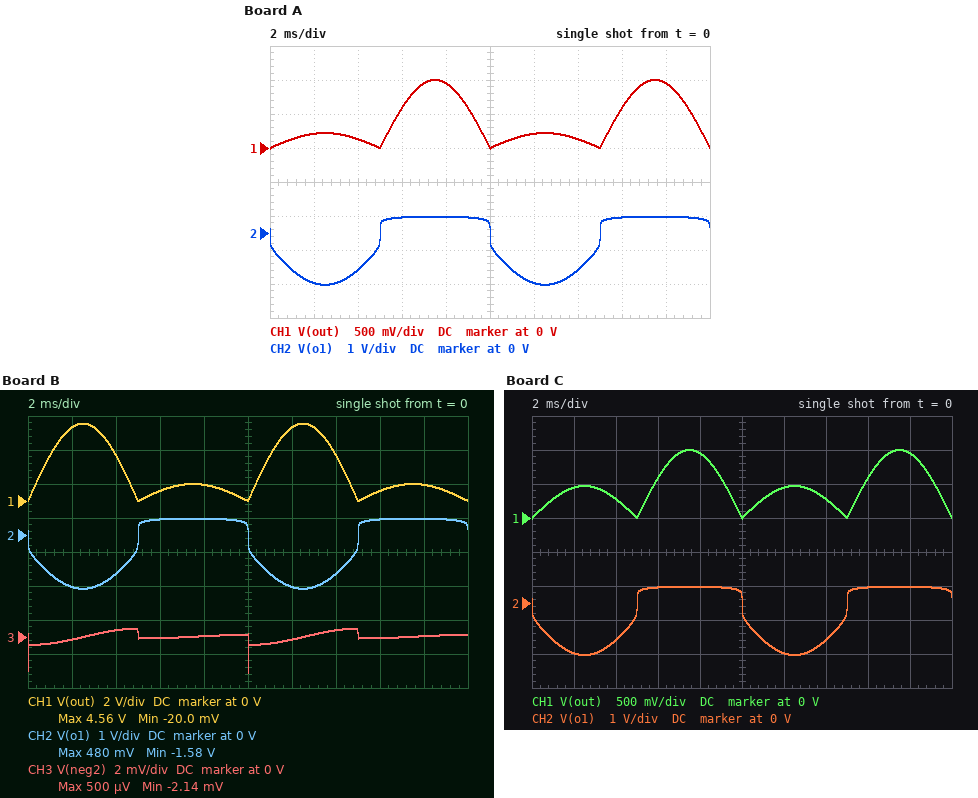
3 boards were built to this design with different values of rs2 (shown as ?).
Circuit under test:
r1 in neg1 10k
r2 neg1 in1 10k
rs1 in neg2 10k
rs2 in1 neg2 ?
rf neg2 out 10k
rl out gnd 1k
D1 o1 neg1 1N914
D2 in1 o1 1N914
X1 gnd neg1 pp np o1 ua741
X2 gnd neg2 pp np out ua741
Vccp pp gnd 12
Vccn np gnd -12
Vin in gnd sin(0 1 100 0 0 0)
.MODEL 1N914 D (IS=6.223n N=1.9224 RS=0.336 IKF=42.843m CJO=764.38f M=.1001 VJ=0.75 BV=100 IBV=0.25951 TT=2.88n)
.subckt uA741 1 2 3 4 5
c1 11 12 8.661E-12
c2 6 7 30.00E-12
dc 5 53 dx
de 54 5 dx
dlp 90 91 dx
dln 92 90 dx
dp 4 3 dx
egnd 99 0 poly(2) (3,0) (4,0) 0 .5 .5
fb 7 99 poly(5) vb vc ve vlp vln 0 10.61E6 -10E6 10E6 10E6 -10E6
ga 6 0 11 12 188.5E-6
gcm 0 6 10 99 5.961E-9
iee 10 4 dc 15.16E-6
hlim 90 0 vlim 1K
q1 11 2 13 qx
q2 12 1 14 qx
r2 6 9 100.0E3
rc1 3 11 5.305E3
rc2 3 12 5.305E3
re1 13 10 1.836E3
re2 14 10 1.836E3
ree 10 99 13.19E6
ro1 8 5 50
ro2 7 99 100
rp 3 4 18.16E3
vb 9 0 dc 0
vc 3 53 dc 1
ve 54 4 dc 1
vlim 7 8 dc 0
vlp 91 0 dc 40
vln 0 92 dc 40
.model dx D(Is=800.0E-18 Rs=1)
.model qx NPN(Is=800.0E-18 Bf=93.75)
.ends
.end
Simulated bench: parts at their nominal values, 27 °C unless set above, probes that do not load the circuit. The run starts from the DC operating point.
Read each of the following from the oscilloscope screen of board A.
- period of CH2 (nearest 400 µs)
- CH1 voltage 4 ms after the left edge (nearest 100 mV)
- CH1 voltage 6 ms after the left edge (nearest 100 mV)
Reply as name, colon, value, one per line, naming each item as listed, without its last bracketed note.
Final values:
period of CH2: 10.0 ms
CH1 voltage 4 ms after the left edge: 100 mV
CH1 voltage 6 ms after the left edge: 600 mV
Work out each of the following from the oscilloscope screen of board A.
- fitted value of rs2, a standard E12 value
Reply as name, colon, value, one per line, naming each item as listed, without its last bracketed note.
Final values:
fitted value of rs2, a standard E12 value: 8.2 kΩ
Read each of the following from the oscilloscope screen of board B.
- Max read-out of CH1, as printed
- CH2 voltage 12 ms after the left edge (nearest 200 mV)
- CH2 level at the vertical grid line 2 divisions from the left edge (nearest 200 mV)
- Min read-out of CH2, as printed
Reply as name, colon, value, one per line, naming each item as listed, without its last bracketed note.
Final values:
Max read-out of CH1, as printed: 4.56 V
CH2 voltage 12 ms after the left edge: -1.6 V
CH2 level at the vertical grid line 2 divisions from the left edge: -1.2 V
Min read-out of CH2, as printed: -1.58 V
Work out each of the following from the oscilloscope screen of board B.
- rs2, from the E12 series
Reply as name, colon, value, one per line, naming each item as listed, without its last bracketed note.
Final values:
rs2, from the E12 series: 1.8 kΩ
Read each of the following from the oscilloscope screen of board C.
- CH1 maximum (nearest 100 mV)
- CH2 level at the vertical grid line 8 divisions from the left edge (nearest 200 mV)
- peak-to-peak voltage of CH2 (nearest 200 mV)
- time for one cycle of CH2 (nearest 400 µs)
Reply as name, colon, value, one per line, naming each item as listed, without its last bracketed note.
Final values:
CH1 maximum: 1.0 V
CH2 level at the vertical grid line 8 divisions from the left edge: 400 mV
peak-to-peak voltage of CH2: 2.0 V
time for one cycle of CH2: 10.0 ms
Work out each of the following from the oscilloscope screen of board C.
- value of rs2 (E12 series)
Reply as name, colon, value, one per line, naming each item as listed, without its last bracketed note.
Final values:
value of rs2: 6.8 kΩ
